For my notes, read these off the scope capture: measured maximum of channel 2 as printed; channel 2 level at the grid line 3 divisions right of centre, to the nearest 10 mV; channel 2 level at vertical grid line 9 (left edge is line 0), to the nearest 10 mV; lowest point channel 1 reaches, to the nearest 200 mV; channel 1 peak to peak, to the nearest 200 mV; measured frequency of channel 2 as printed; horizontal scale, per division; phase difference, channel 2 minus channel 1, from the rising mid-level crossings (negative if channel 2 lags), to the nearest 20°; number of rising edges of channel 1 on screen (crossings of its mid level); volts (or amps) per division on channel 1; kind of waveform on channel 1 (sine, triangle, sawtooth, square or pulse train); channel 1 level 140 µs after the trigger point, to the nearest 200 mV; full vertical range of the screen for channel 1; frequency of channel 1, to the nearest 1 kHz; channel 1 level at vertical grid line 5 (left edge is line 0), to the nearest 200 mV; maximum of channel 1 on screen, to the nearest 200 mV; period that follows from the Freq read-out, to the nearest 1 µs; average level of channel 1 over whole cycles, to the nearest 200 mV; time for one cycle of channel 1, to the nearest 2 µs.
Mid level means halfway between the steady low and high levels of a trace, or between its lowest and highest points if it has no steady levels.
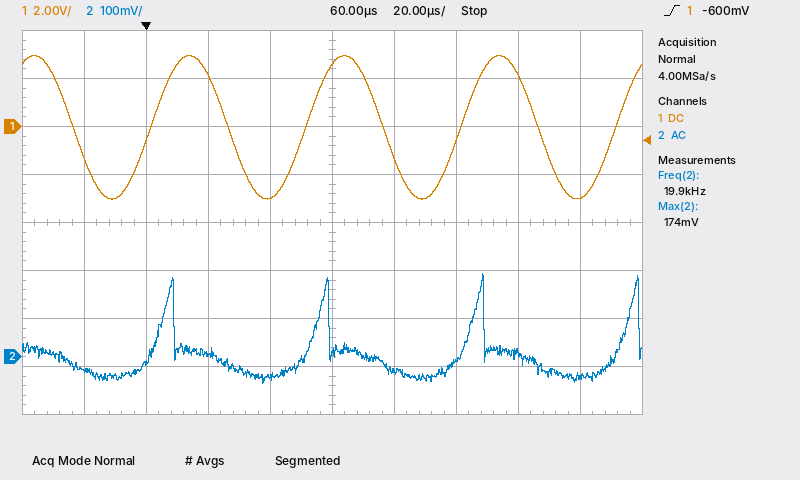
174 mV
10 mV
-40 mV
-3.0 V
6.0 V
19.9 kHz
20 µs
-20°
4
2 V
sine
-3.0 V
16 V
20 kHz
2.6 V
3.0 V
50 µs
0.0 V
50 µs
